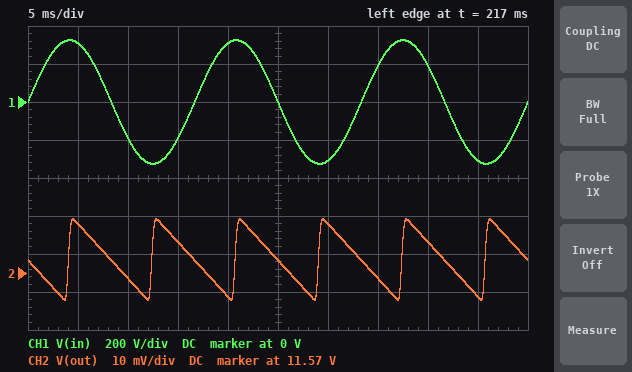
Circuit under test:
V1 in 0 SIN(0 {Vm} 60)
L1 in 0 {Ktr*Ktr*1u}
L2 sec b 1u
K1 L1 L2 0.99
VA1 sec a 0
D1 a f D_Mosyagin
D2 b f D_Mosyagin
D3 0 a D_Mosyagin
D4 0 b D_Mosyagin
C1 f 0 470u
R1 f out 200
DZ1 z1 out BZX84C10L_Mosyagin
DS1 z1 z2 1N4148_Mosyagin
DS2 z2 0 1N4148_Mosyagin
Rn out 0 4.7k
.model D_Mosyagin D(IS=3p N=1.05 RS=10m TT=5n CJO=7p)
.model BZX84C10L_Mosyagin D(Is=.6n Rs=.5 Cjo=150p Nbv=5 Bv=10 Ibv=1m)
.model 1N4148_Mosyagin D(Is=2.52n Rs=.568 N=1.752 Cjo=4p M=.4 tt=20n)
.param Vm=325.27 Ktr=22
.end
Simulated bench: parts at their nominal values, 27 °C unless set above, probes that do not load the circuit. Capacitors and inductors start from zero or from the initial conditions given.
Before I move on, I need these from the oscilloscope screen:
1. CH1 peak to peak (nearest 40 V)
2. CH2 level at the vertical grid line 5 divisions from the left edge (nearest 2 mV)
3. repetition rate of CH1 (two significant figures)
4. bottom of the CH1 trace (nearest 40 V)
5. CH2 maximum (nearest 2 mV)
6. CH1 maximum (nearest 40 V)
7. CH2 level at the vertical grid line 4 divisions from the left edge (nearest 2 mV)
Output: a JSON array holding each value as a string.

["640 V", "11.574 V", "60 Hz", "-320 V", "11.584 V", "320 V", "11.564 V"]
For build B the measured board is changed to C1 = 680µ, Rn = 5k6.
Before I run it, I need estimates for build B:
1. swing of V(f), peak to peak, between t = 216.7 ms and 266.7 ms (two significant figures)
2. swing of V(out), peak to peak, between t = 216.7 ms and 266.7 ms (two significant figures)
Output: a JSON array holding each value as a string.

["92 mV", "14 mV"]
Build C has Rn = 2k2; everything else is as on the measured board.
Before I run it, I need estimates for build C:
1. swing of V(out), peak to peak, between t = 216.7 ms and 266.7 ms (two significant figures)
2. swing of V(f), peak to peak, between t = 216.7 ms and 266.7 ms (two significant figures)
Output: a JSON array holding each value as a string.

["32 mV", "140 mV"]
